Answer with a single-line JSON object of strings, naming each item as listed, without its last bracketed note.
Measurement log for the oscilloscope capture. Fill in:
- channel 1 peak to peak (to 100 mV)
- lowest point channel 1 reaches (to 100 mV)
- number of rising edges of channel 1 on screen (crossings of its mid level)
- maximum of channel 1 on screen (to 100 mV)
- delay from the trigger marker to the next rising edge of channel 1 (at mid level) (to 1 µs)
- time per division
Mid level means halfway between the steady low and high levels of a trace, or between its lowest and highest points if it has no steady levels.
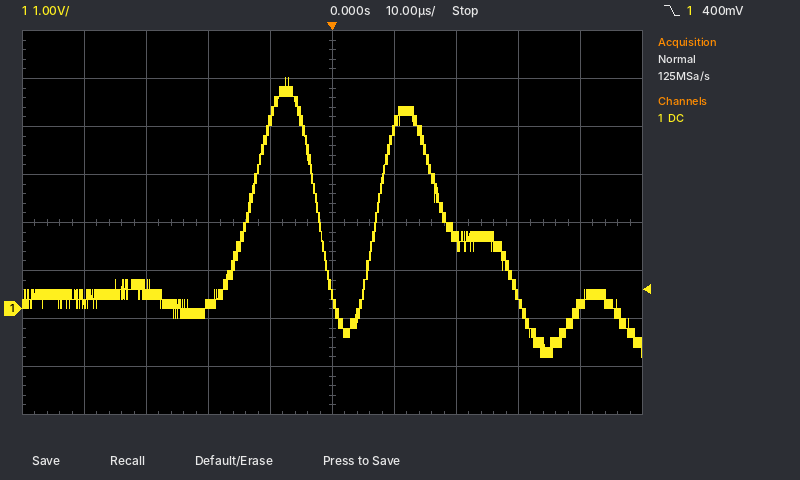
{"channel 1 peak to peak": "5.8 V", "lowest point channel 1 reaches": "-1.0 V", "number of rising edges of channel 1 on screen": "2", "maximum of channel 1 on screen": "4.8 V", "delay from the trigger marker to the next rising edge of channel 1 (at mid level)": "7 µs", "time per division": "10 µs"}
